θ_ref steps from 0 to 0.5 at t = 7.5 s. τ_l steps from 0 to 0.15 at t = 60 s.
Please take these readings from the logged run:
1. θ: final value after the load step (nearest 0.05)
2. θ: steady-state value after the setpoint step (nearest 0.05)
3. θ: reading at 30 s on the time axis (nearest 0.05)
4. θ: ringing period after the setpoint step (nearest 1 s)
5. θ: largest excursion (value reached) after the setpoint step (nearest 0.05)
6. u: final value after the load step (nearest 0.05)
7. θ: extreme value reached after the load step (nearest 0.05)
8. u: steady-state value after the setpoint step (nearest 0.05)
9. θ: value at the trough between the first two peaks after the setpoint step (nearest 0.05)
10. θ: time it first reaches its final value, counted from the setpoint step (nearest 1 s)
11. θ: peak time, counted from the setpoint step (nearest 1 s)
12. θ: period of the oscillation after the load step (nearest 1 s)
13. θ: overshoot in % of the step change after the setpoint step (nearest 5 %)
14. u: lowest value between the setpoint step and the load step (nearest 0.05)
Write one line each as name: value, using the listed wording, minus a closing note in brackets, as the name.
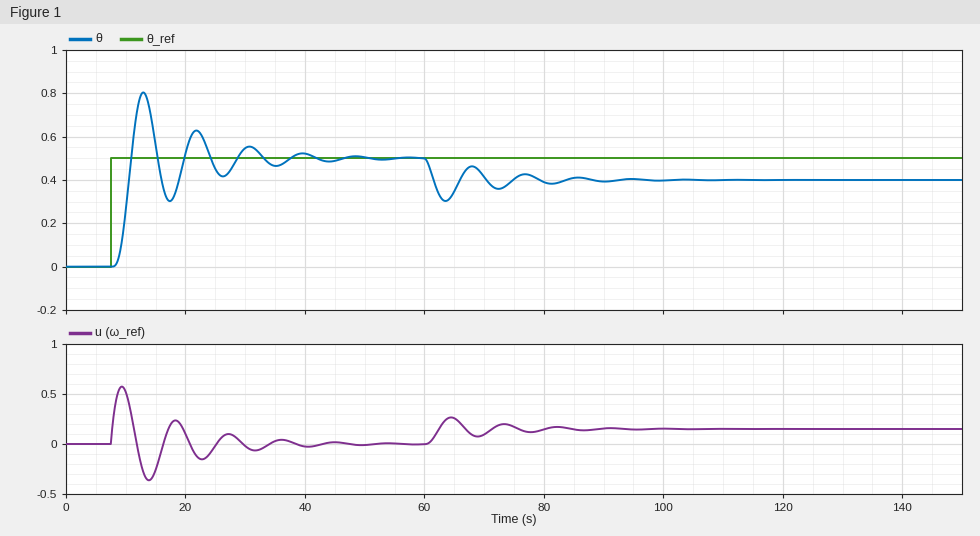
θ: final value after the load step: 0.40
θ: steady-state value after the setpoint step: 0.50
θ: reading at 30 s on the time axis: 0.55
θ: ringing period after the setpoint step: 9 s
θ: largest excursion (value reached) after the setpoint step: 0.80
u: final value after the load step: 0.15
θ: extreme value reached after the load step: 0.30
u: steady-state value after the setpoint step: 0.00
θ: value at the trough between the first two peaks after the setpoint step: 0.30
θ: time it first reaches its final value, counted from the setpoint step: 3 s
θ: peak time, counted from the setpoint step: 5 s
θ: period of the oscillation after the load step: 9 s
θ: overshoot in % of the step change after the setpoint step: 60 %
u: lowest value between the setpoint step and the load step: -0.35
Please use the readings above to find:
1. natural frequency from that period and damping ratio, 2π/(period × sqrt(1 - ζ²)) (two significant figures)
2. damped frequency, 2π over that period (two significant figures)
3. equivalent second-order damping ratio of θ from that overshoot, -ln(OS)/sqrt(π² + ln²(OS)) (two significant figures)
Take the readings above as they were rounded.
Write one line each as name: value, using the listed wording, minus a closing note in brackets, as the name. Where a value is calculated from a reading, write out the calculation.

natural frequency from that period and damping ratio, 2π/(period × sqrt(1 - ζ²)): 2π / (9 × sqrt(1 - 0.16²)) = 0.71 rad/s
damped frequency, 2π over that period: 2π / 9 = 0.70 rad/s
equivalent second-order damping ratio of θ from that overshoot, -ln(OS)/sqrt(π² + ln²(OS)): ln(0.6) = -0.511; 0.511 / sqrt(9.870 + 0.261) = 0.16
